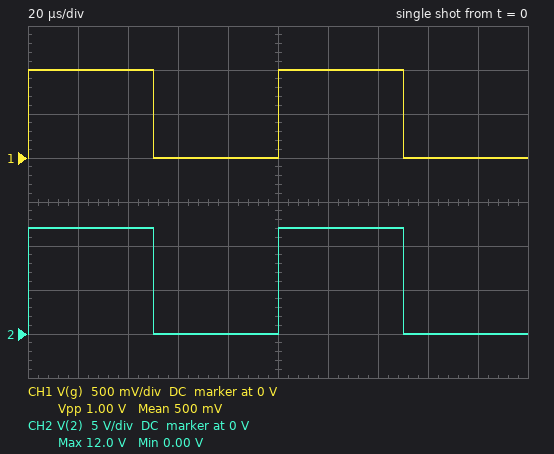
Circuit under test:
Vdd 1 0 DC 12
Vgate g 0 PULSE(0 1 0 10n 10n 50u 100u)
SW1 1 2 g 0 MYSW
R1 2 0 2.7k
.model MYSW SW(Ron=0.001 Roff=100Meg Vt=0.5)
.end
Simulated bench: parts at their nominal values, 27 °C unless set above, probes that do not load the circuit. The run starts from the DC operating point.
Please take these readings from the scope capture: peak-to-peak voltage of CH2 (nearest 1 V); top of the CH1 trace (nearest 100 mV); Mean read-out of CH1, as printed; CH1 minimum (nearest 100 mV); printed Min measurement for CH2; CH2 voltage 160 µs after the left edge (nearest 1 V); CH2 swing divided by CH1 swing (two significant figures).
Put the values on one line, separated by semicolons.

12 V; 1.0 V; 500 mV; 0 V; 0.00 V; 0 V; 12
